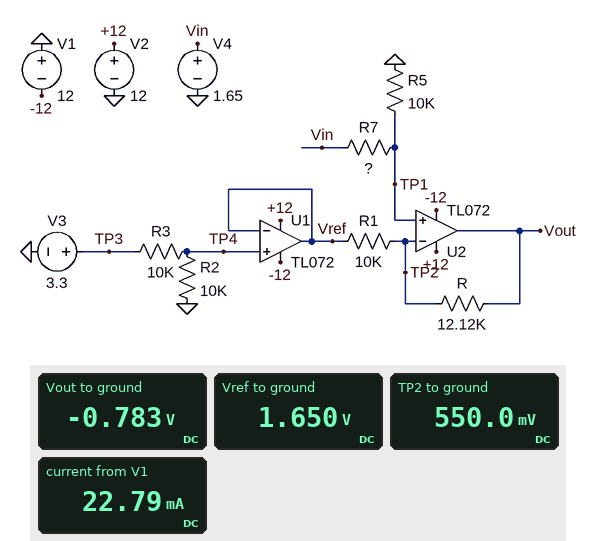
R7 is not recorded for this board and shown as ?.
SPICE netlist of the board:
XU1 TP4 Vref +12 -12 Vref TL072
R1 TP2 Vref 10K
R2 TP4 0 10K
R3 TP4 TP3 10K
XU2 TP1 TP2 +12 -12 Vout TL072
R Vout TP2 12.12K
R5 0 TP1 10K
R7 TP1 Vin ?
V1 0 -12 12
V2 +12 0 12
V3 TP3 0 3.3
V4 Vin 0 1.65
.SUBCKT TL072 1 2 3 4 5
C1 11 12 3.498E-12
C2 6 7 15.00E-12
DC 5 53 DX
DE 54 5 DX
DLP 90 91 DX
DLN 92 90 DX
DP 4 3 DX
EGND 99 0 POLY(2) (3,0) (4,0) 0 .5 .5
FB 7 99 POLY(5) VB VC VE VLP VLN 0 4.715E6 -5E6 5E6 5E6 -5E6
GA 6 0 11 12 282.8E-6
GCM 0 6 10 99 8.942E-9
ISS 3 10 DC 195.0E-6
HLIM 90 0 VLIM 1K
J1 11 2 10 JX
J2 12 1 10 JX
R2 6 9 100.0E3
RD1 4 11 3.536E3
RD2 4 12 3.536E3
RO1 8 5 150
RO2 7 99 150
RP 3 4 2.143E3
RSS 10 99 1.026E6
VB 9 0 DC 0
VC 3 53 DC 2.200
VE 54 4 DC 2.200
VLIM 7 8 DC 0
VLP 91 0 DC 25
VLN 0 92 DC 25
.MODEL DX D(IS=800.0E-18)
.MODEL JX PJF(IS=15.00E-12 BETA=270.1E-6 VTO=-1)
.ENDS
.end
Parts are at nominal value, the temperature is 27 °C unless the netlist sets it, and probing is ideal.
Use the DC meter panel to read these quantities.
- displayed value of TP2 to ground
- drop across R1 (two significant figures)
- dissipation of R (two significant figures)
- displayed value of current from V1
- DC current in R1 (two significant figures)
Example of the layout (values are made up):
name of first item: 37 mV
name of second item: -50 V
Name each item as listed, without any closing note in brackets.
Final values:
displayed value of TP2 to ground: 550.0 mV
drop across R1: 1.1 V
dissipation of R: 150 µW
displayed value of current from V1: 22.79 mA
DC current in R1: 110 µA
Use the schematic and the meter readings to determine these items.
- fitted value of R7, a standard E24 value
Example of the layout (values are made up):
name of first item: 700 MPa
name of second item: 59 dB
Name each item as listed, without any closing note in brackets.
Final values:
fitted value of R7, a standard E24 value: 20 kΩ
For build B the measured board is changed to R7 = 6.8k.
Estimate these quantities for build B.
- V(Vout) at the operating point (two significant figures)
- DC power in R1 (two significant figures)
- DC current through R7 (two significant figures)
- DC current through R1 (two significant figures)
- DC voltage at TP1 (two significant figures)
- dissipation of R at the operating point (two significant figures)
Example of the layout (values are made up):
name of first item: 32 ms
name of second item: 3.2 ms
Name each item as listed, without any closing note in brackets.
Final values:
V(Vout) at the operating point: 170 mV
DC power in R1: 45 µW
DC current through R7: 98 µA
DC current through R1: 67 µA
DC voltage at TP1: 980 mV
dissipation of R at the operating point: 54 µW
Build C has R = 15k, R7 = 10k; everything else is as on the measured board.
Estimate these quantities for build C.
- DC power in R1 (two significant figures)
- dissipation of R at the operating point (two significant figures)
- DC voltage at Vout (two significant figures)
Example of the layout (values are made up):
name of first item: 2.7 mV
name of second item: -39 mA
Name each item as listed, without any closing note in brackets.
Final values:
DC power in R1: 68 µW
dissipation of R at the operating point: 100 µW
DC voltage at Vout: -410 mV
